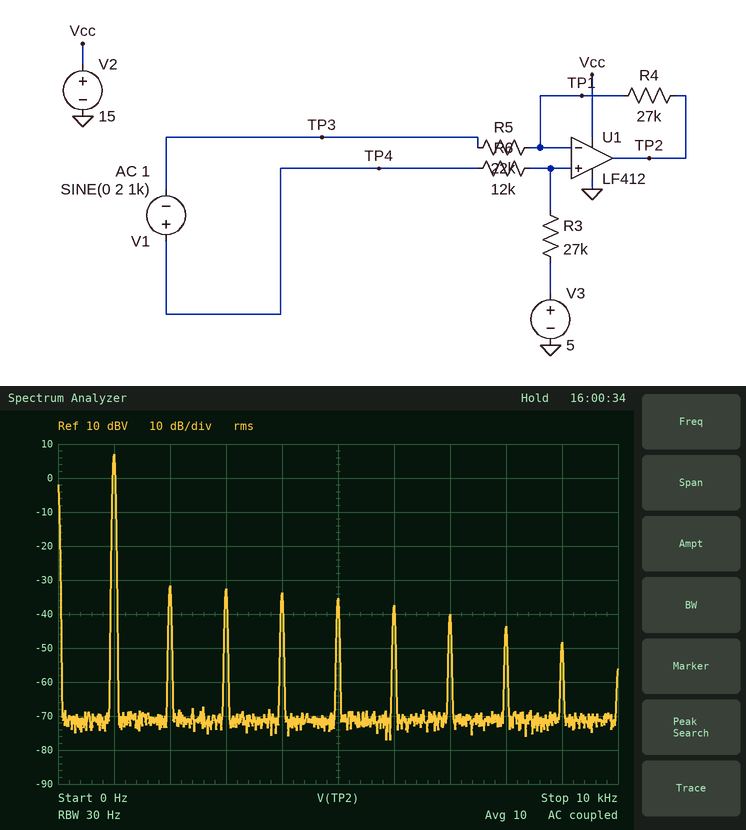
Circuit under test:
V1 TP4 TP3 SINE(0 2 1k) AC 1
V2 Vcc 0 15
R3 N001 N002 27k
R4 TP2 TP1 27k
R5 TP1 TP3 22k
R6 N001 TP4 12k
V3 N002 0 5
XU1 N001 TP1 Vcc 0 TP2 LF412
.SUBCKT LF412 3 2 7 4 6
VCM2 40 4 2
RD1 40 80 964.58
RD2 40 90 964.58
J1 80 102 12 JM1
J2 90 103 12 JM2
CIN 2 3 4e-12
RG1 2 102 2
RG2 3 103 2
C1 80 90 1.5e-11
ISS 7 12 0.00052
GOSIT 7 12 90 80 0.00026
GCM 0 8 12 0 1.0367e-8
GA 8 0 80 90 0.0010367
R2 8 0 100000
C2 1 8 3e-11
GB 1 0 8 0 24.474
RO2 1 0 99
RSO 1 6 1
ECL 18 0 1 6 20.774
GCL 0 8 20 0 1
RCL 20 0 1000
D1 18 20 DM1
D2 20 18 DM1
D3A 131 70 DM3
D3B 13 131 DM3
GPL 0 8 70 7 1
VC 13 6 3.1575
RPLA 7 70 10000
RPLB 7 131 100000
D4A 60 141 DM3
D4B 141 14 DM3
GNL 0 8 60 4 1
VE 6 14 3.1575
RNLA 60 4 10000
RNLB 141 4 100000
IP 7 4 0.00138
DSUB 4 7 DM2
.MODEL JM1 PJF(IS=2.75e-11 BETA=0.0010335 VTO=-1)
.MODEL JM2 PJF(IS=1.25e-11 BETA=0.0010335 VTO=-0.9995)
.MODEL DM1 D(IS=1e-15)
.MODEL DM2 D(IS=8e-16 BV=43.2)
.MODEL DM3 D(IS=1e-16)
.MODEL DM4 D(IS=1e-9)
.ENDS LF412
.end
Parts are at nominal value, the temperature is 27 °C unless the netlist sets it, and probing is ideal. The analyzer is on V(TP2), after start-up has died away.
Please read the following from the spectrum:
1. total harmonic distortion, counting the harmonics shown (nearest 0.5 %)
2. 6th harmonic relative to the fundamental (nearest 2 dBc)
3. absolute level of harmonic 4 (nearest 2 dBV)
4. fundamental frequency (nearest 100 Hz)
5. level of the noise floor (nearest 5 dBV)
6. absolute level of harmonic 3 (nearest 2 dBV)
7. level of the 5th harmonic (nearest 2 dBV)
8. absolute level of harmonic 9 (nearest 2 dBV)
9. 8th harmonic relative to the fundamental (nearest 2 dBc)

2.0 %
-44 dBc
-34 dBV
1.0 kHz
-70 dBV
-32 dBV
-36 dBV
-48 dBV
-50 dBc
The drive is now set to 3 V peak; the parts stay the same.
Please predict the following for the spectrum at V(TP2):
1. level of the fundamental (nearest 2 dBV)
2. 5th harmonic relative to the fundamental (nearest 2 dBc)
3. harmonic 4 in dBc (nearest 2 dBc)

10 dBV
-56 dBc
-30 dBc
